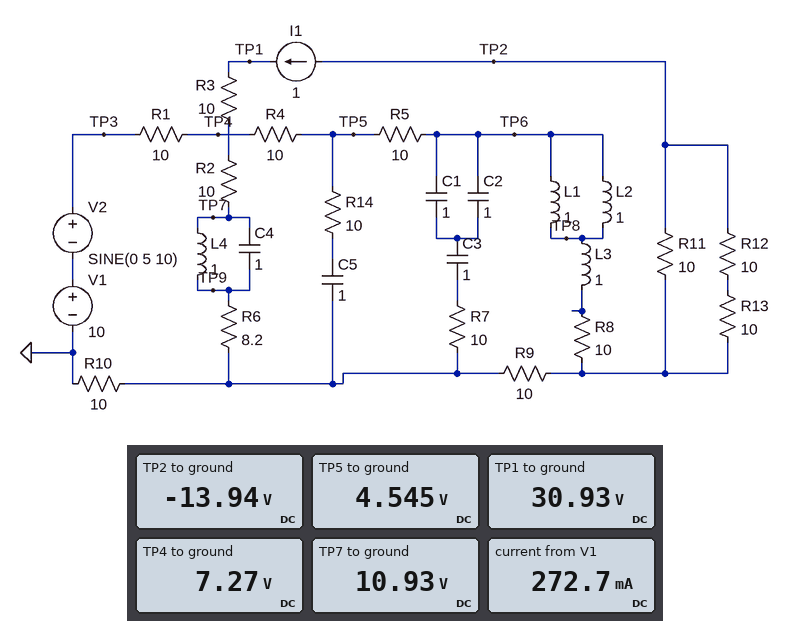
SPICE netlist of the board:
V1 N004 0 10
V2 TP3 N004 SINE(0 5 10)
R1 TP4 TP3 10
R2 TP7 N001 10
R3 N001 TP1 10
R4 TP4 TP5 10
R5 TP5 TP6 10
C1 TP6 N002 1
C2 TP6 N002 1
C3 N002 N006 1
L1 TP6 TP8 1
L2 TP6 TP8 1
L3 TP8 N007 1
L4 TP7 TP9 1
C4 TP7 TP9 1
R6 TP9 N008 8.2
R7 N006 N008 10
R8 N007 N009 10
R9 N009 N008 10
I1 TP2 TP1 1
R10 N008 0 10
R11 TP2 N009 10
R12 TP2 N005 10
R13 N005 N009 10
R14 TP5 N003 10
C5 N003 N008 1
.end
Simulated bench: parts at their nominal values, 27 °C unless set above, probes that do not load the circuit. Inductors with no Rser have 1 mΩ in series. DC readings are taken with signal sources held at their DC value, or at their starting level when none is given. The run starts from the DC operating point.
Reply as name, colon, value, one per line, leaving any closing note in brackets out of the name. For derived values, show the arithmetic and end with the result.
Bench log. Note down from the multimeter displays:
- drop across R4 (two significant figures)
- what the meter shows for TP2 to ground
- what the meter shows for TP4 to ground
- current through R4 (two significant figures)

drop across R4: 7.27 V - 4.545 V = 2.7 V
what the meter shows for TP2 to ground: -13.94 V
what the meter shows for TP4 to ground: 7.27 V
current through R4: (7.27 V - 4.545 V) / 10 Ω = 270 mA
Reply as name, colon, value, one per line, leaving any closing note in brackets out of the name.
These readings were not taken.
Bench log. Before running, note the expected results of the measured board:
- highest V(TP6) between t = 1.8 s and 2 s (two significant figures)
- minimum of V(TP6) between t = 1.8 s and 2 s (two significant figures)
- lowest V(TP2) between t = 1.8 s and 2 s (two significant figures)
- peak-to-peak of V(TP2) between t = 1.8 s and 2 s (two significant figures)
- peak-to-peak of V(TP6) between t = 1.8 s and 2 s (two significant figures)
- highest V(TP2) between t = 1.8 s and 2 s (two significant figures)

highest V(TP6) between t = 1.8 s and 2 s: 1.8 V
minimum of V(TP6) between t = 1.8 s and 2 s: -1.8 V
lowest V(TP2) between t = 1.8 s and 2 s: -11 V
peak-to-peak of V(TP2) between t = 1.8 s and 2 s: 2.8 V
peak-to-peak of V(TP6) between t = 1.8 s and 2 s: 3.6 V
highest V(TP2) between t = 1.8 s and 2 s: -8.6 V
